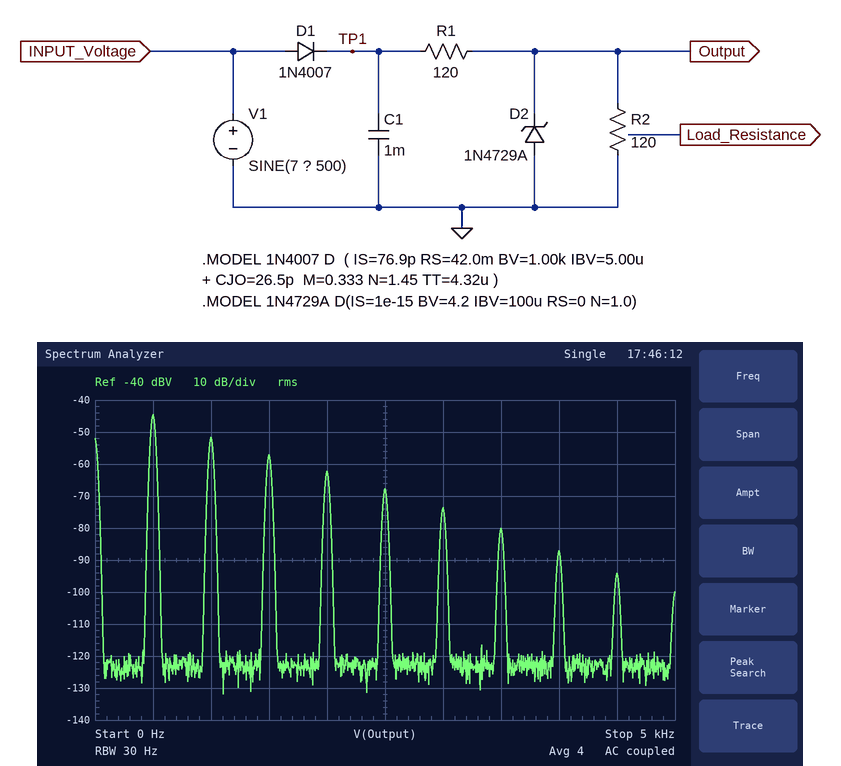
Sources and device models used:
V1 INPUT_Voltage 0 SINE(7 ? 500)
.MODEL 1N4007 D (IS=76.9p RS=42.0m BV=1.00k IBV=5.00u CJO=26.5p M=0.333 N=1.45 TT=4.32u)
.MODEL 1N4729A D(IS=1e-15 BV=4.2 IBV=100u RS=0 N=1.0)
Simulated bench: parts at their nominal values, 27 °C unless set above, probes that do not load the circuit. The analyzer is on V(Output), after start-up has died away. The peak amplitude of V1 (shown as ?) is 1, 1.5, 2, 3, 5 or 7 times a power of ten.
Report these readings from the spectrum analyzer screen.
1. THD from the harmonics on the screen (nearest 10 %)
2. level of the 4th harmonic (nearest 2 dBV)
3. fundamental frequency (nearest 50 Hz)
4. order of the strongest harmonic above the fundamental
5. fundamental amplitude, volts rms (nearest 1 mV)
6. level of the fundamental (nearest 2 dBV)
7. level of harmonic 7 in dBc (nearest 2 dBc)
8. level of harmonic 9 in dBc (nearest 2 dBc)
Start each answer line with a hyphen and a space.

- 50 %
- -62 dBV
- 500 Hz
- 2
- 6 mV
- -44 dBV
- -36 dBc
- -50 dBc
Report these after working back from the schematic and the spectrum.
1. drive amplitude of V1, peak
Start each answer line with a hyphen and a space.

- 500 mV
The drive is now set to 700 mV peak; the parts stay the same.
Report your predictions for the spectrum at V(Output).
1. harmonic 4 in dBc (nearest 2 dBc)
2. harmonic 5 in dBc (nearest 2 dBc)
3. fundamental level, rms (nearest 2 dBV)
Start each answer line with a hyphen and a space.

- -16 dBc
- -20 dBc
- -44 dBV
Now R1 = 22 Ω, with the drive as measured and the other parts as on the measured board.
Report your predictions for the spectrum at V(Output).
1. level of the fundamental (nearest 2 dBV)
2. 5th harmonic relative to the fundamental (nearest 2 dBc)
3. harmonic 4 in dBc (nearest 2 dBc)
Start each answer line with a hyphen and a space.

- -62 dBV
- -26 dBc
- -20 dBc
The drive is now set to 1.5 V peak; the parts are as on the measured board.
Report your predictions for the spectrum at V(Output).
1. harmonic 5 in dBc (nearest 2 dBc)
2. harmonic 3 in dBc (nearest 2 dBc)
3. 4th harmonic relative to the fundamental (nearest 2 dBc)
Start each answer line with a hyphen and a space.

- -18 dBc
- -10 dBc
- -14 dBc
